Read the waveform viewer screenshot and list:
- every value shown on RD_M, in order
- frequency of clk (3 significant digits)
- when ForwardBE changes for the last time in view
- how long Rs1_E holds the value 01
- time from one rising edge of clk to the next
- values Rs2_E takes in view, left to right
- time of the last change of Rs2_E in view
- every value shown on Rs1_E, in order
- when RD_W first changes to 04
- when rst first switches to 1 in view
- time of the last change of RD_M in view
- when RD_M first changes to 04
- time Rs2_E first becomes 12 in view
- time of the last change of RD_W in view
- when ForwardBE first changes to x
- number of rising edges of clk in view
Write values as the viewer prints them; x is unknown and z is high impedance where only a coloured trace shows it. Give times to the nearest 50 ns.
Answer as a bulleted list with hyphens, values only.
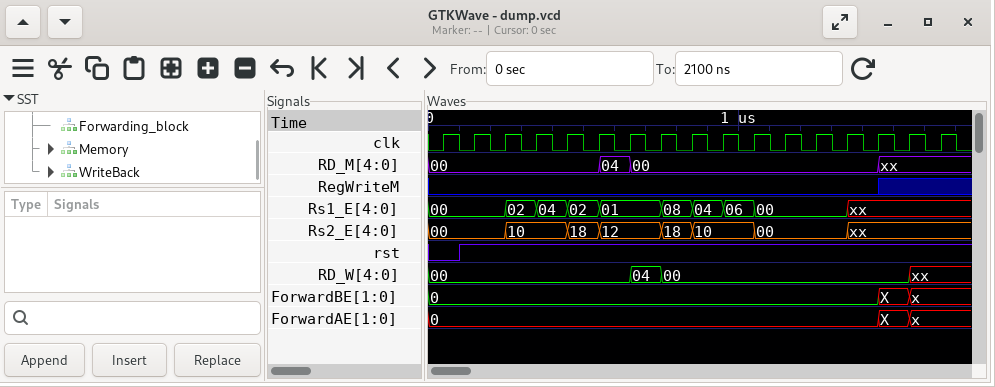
- 00, 04, 00, xx
- 10.0 MHz
- 1550 ns
- 200 ns
- 100 ns
- 00, 10, 18, 12, 18, 10, 00, xx
- 1350 ns
- 00, 02, 04, 02, 01, 08, 04, 06, 00, xx
- 650 ns
- 100 ns
- 1450 ns
- 550 ns
- 550 ns
- 1550 ns
- 1550 ns
- 17
